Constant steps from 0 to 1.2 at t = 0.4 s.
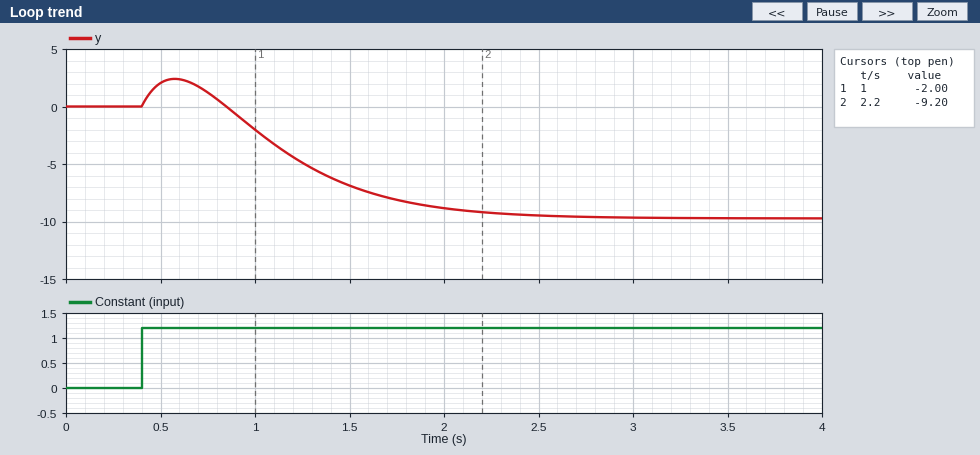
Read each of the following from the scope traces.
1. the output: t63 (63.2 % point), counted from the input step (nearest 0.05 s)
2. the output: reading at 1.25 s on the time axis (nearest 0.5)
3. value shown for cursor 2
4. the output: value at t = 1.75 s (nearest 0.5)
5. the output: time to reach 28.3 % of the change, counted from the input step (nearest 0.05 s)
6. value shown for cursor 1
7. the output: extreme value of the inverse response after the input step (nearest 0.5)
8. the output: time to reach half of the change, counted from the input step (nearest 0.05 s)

1.00 s
-5.0
-9.20
-8.0
0.65 s
-2.00
2.5
0.85 s
